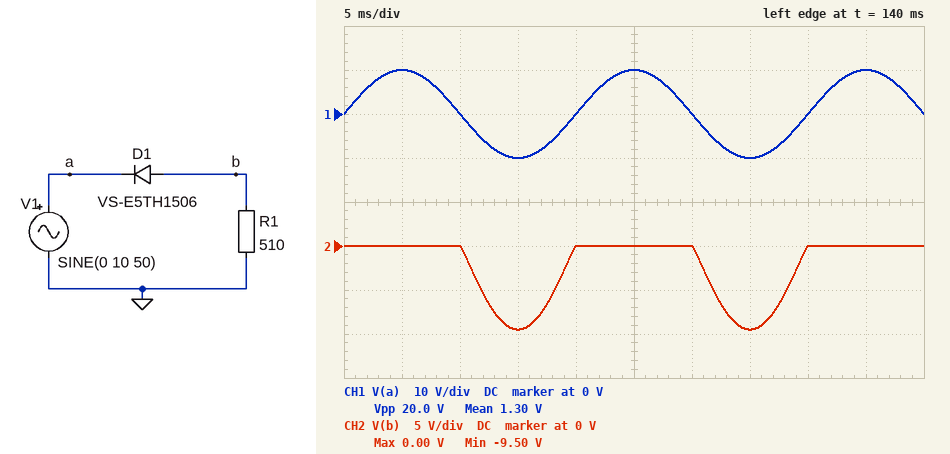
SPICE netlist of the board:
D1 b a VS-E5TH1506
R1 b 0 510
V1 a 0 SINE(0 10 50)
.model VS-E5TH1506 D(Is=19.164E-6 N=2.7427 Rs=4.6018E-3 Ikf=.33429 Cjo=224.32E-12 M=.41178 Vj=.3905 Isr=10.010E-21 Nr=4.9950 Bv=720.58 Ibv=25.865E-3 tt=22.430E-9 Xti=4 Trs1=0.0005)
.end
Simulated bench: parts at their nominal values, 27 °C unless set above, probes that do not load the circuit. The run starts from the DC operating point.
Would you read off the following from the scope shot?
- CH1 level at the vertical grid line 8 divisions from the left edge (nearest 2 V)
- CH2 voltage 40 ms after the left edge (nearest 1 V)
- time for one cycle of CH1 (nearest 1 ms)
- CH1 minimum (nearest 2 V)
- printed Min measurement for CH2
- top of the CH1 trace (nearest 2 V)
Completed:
0 V
0 V
20 ms
-10 V
-9.50 V
10 V
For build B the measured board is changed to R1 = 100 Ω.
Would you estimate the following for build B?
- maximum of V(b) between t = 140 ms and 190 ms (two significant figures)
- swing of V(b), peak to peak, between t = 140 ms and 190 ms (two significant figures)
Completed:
2.0 mV
9.4 V
